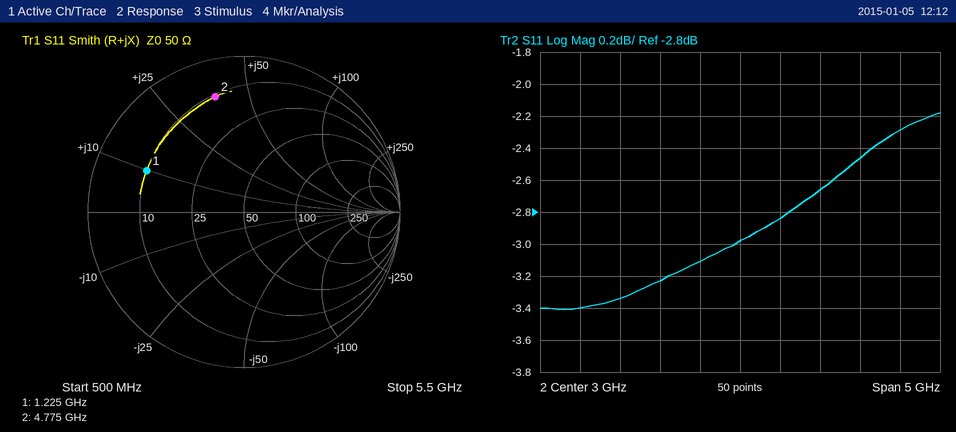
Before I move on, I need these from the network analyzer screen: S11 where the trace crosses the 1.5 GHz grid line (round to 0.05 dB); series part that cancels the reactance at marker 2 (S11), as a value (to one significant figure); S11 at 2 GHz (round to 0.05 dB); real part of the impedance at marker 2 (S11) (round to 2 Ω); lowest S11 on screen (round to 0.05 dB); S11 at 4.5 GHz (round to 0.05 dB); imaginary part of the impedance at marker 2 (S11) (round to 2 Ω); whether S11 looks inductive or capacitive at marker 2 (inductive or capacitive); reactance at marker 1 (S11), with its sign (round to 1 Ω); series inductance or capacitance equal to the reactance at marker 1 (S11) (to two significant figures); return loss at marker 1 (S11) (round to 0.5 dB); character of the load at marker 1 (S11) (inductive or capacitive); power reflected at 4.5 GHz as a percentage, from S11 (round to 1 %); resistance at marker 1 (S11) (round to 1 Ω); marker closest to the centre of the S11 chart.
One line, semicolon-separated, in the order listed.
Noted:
-3.35 dB; 900 fF; -3.25 dB; 10 Ω; -3.40 dB; -2.45 dB; +38 Ω; inductive; +10 Ω; 1.3 nH; 3.5 dB; inductive; 57 %; 10 Ω; marker 1
